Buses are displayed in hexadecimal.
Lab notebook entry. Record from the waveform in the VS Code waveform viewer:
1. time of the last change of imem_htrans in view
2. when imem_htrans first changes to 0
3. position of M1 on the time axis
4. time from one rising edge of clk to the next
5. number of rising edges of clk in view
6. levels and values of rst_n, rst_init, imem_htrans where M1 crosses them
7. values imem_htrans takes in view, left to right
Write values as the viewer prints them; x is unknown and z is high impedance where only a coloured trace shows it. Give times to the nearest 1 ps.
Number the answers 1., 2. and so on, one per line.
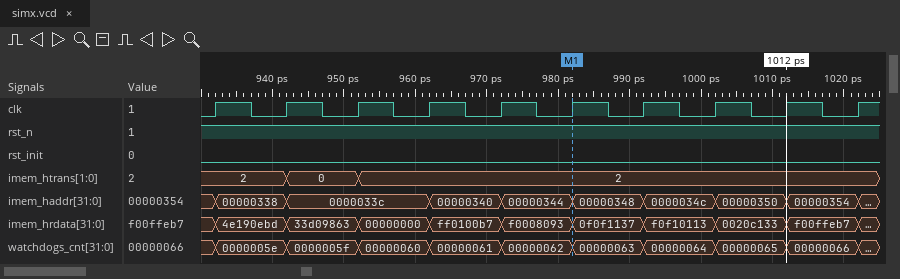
1. 952 ps
2. 942 ps
3. 982 ps
4. 10 ps
5. 10
6. rst_n=1, rst_init=0, imem_htrans=2
7. 2, 0, 2
